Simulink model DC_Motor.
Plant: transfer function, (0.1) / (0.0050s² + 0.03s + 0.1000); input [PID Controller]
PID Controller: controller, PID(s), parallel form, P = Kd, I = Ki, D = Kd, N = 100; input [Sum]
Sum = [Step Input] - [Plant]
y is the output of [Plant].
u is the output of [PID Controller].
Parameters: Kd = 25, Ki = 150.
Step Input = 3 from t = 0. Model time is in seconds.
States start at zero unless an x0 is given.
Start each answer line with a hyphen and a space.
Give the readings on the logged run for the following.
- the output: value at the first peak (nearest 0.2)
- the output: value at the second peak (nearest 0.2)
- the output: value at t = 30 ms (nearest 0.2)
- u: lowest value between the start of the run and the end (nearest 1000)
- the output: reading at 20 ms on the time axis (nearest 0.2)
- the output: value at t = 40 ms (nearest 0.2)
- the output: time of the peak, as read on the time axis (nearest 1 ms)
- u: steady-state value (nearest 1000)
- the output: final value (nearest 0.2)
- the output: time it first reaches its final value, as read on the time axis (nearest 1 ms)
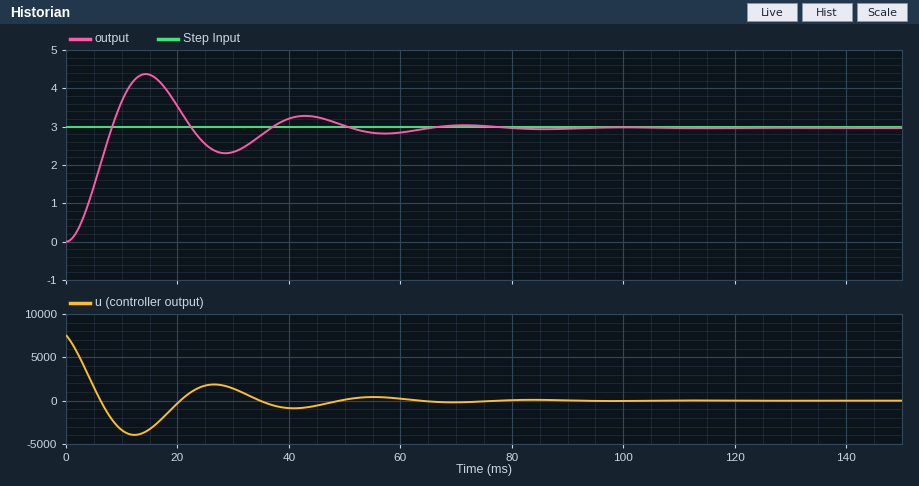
- 4.4
- 3.2
- 2.4
- -4000
- 3.6
- 3.2
- 14 ms
- 0
- 3.0
- 8 ms
